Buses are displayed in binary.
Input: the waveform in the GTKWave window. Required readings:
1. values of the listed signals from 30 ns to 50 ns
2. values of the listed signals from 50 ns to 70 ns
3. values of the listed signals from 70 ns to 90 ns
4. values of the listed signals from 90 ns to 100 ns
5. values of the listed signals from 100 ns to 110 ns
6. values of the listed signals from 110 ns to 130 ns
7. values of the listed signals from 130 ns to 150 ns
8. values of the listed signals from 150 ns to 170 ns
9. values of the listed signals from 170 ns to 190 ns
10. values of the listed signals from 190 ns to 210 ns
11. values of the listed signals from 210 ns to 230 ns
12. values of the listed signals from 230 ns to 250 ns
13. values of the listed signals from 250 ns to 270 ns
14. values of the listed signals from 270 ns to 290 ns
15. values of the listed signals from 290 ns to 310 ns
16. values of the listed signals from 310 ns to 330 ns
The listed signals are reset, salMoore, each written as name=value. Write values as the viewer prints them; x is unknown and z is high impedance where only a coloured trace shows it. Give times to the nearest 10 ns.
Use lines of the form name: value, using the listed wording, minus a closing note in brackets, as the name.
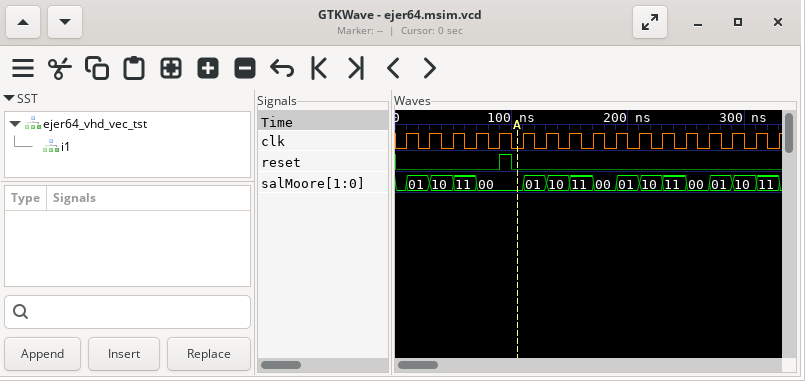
values of the listed signals from 30 ns to 50 ns: reset=0, salMoore=10
values of the listed signals from 50 ns to 70 ns: reset=0, salMoore=11
values of the listed signals from 70 ns to 90 ns: reset=0, salMoore=00
values of the listed signals from 90 ns to 100 ns: reset=1, salMoore=00
values of the listed signals from 100 ns to 110 ns: reset=0, salMoore=00
values of the listed signals from 110 ns to 130 ns: reset=0, salMoore=01
values of the listed signals from 130 ns to 150 ns: reset=0, salMoore=10
values of the listed signals from 150 ns to 170 ns: reset=0, salMoore=11
values of the listed signals from 170 ns to 190 ns: reset=0, salMoore=00
values of the listed signals from 190 ns to 210 ns: reset=0, salMoore=01
values of the listed signals from 210 ns to 230 ns: reset=0, salMoore=10
values of the listed signals from 230 ns to 250 ns: reset=0, salMoore=11
values of the listed signals from 250 ns to 270 ns: reset=0, salMoore=00
values of the listed signals from 270 ns to 290 ns: reset=0, salMoore=01
values of the listed signals from 290 ns to 310 ns: reset=0, salMoore=10
values of the listed signals from 310 ns to 330 ns: reset=0, salMoore=11
